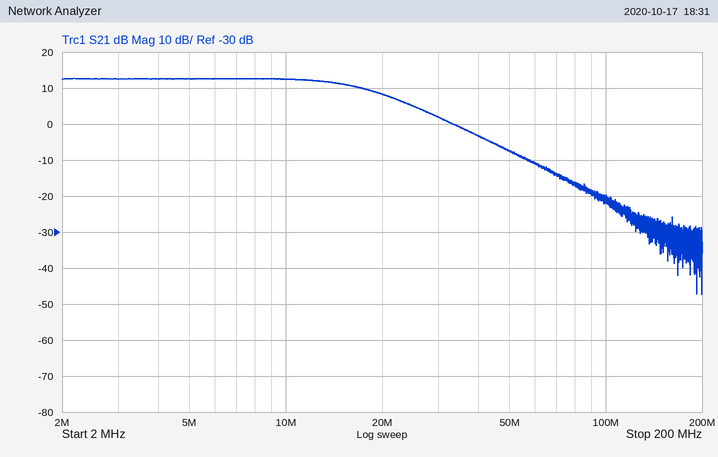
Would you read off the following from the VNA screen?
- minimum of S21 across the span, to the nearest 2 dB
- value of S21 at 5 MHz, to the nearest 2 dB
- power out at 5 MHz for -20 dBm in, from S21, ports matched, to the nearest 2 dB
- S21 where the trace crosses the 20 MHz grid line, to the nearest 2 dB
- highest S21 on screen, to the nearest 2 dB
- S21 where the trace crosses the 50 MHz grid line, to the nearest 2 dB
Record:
-48 dB
12 dB
-8 dBm
8 dB
12 dB
-8 dB
